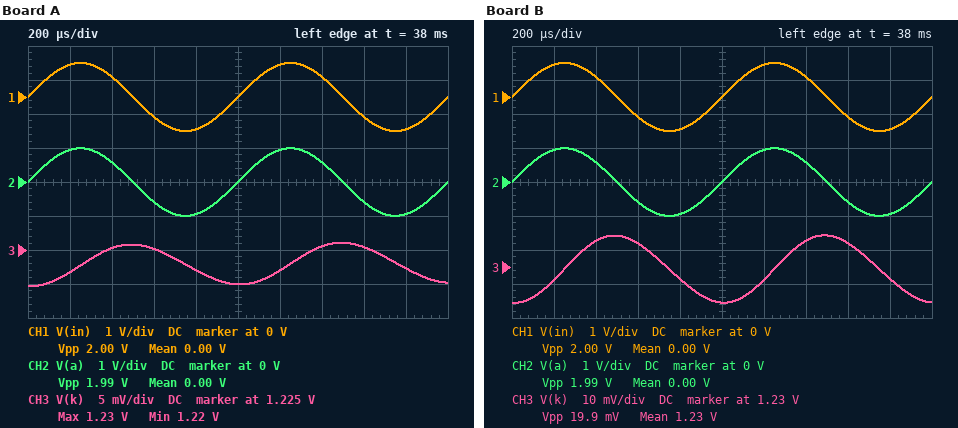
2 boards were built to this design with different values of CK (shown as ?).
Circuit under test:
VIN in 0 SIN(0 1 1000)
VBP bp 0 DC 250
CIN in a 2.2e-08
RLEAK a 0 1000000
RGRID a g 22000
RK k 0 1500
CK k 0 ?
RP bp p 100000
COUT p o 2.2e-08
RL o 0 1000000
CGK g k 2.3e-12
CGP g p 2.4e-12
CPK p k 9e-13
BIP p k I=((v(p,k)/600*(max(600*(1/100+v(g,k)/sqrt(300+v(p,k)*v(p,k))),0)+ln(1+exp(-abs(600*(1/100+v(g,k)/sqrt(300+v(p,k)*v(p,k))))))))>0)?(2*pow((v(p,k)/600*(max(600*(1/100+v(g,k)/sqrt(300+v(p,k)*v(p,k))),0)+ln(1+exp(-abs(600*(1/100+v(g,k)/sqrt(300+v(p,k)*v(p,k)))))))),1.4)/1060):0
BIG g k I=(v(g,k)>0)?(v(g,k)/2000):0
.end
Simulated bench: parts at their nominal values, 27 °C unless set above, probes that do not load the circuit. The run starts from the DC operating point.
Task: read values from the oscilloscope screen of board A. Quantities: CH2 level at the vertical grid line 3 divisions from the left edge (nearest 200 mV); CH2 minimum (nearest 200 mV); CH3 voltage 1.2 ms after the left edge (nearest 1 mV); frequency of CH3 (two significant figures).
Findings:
-600 mV
-1.0 V
1.222 V
1.0 kHz
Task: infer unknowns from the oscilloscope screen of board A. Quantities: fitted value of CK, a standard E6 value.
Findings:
33 µF
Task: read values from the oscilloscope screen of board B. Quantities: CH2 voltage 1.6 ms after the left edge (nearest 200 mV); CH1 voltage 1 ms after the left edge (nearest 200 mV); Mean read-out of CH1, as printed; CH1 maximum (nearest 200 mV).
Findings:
-600 mV
0 V
0.00 V
1.0 V
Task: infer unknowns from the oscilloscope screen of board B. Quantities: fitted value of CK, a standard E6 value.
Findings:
10 µF
